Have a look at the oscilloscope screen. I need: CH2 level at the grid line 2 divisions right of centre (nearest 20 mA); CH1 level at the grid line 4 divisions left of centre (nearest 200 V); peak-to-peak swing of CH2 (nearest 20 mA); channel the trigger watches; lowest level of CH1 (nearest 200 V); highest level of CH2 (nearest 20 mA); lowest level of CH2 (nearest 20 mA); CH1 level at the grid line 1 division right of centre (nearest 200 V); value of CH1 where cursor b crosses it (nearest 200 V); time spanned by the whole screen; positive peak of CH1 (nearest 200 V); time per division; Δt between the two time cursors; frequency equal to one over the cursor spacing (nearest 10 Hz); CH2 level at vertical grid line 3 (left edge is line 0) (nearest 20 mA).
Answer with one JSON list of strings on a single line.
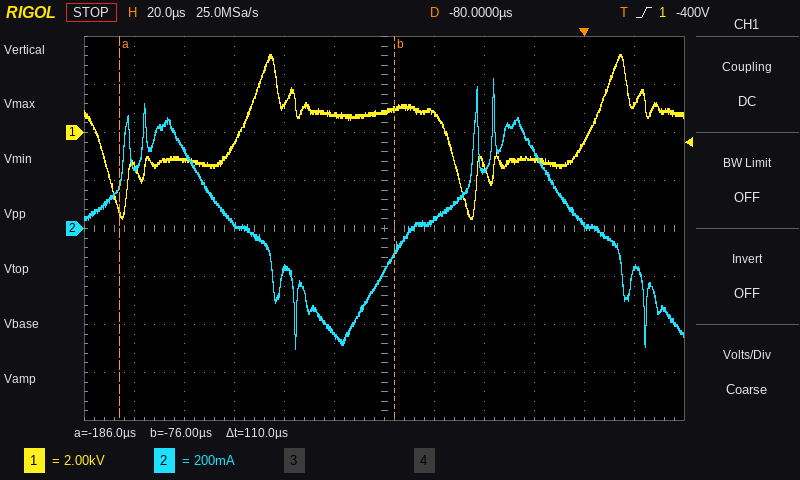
["240 mA", "-1.2 kV", "1.12 A", "CH1", "-3.6 kV", "620 mA", "-500 mA", "800 V", "1.0 kV", "240 µs", "3.2 kV", "20 µs", "110 µs", "9.09 kHz", "20 mA"]
